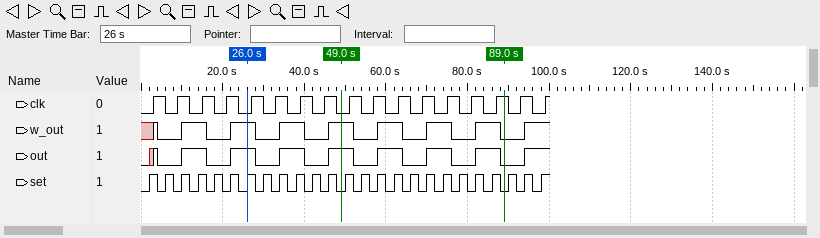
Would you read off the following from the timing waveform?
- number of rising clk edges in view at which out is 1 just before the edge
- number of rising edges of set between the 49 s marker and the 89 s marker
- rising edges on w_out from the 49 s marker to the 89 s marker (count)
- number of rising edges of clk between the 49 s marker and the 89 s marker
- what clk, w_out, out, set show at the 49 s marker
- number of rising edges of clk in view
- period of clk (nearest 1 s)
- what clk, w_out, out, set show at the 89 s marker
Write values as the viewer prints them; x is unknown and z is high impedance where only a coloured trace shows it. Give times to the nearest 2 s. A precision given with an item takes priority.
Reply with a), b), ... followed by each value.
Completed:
a) 8
b) 10
c) 3
d) 7
e) clk=0, w_out=1, out=1, set=0
f) 17
g) 6 s
h) clk=1, w_out=0, out=0, set=0
